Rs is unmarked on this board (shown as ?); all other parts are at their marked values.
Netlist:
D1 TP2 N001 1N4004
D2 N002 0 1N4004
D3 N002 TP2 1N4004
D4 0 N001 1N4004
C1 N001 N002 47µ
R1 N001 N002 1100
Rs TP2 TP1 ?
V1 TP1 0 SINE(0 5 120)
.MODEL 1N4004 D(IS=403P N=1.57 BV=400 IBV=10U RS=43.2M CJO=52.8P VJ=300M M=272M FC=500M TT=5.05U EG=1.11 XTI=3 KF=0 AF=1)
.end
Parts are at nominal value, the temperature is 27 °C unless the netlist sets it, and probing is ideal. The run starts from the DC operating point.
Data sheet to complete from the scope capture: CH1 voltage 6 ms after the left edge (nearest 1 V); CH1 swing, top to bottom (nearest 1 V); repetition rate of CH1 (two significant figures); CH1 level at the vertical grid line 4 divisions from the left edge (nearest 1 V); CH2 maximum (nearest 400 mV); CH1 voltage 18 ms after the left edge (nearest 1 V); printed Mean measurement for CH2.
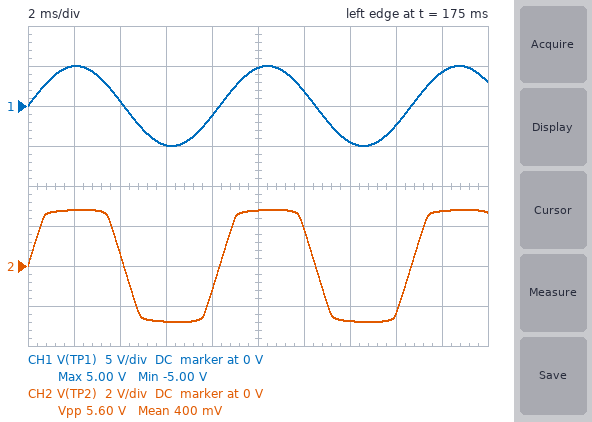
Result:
-5 V
10 V
120 Hz
-1 V
2.8 V
4 V
400 mV
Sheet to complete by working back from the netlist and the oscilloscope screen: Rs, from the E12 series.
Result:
680 Ω
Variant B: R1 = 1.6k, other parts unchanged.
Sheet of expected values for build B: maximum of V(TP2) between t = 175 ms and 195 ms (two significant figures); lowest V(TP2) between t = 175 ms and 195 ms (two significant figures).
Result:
3.1 V
-3.1 V
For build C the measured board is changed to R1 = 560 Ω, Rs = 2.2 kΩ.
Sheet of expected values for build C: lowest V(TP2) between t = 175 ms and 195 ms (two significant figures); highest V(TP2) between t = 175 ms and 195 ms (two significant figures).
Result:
-1.7 V
1.7 V
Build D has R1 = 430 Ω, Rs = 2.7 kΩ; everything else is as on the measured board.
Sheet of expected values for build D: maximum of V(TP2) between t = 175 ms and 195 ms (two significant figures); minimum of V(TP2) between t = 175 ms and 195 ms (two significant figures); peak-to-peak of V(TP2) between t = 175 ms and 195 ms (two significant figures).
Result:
1.5 V
-1.5 V
3.0 V
